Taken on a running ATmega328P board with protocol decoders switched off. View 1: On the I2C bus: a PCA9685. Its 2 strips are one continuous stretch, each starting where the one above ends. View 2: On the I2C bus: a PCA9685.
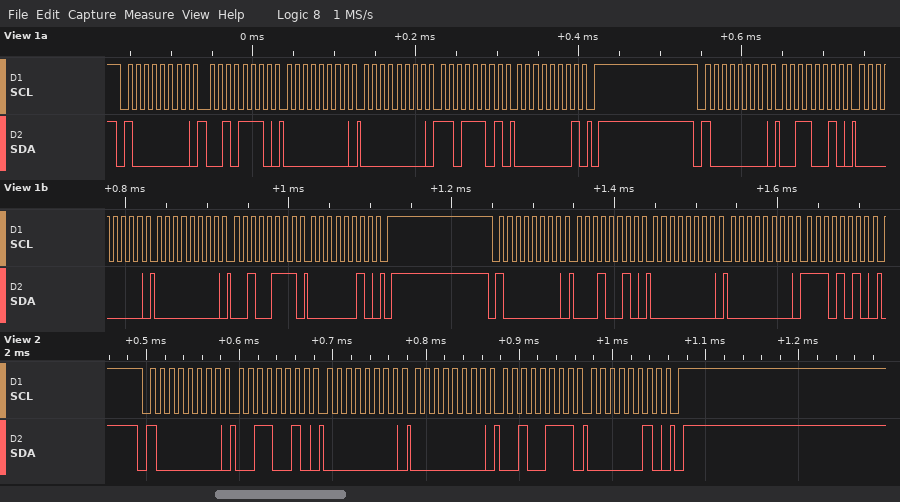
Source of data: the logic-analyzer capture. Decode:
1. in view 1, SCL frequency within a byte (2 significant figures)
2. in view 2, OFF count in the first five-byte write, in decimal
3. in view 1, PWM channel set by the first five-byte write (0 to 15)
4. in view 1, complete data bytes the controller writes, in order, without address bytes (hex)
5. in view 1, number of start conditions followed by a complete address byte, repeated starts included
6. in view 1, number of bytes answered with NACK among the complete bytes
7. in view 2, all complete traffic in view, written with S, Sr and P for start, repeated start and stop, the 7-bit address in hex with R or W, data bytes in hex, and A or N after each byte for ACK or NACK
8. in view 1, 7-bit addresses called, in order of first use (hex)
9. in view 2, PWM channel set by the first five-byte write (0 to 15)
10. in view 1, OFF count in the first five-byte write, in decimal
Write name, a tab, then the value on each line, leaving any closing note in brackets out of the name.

in view 1, SCL frequency within a byte	100 kHz
in view 2, OFF count in the first five-byte write, in decimal	551
in view 1, PWM channel set by the first five-byte write	10
in view 1, complete data bytes the controller writes, in order, without address bytes	2E 00 00 DD 01 32 00 00 27 02 12 00 00 EA
in view 1, number of start conditions followed by a complete address byte, repeated starts included	3
in view 1, number of bytes answered with NACK among the complete bytes	0
in view 2, all complete traffic in view, written with S, Sr and P for start, repeated start and stop, the 7-bit address in hex with R or W, data bytes in hex, and A or N after each byte for ACK or NACK	S 40W A 32 A 00 A 00 A 27 A 02 A P
in view 1, 7-bit addresses called, in order of first use	0x40
in view 2, PWM channel set by the first five-byte write	11
in view 1, OFF count in the first five-byte write, in decimal	477
